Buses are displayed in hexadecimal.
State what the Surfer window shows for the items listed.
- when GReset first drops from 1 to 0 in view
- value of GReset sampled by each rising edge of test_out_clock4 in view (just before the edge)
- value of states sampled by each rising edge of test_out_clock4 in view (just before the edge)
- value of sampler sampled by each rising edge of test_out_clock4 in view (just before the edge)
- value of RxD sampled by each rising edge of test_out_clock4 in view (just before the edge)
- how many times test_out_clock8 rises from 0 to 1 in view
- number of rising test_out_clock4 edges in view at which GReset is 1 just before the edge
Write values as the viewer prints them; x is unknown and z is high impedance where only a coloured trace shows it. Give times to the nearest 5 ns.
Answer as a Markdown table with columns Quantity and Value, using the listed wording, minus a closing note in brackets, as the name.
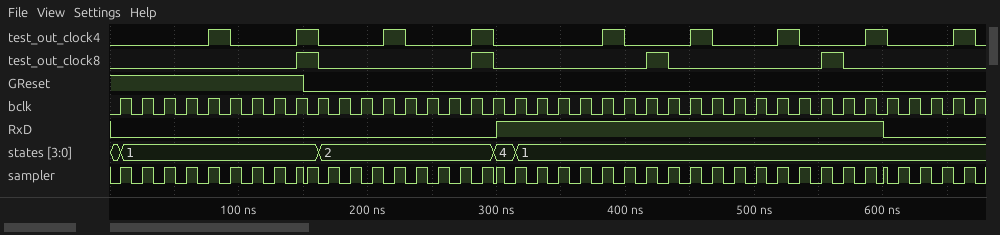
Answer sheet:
| Quantity | Value |
|---|---|
| when GReset first drops from 1 to 0 in view | 150 ns |
| value of GReset sampled by each rising edge of test_out_clock4 in view | 1 1 0 0 0 0 0 0 0 |
| value of states sampled by each rising edge of test_out_clock4 in view | 1, 1, 2, 2, 1, 1, 1, 1, 1 |
| value of sampler sampled by each rising edge of test_out_clock4 in view | 0 0 1 1 0 0 0 0 1 |
| value of RxD sampled by each rising edge of test_out_clock4 in view | 0 0 0 0 1 1 1 1 0 |
| how many times test_out_clock8 rises from 0 to 1 in view | 4 |
| number of rising test_out_clock4 edges in view at which GReset is 1 just before the edge | 2 |
